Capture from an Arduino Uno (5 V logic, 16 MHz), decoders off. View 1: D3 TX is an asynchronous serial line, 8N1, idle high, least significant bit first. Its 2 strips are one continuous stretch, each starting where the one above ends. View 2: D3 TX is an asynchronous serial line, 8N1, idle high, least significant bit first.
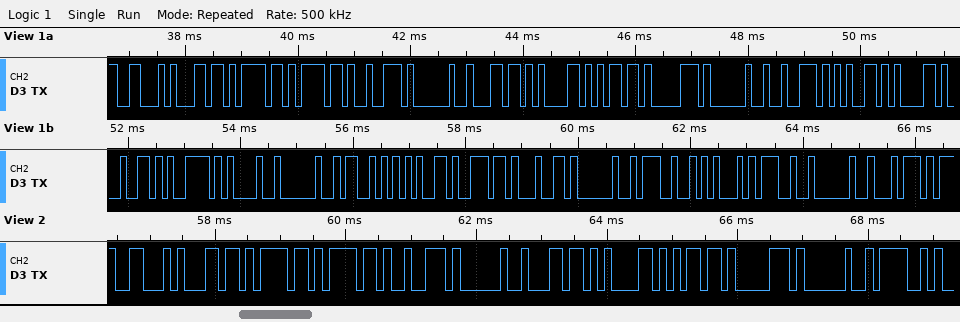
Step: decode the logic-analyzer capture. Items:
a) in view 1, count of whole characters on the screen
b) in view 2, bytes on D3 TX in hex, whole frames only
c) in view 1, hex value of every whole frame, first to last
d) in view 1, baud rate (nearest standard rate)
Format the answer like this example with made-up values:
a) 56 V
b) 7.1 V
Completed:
a) 28
b) 46 6C 6F 6F 72 20 6C 61 6D 70 20 4F
c) 46 6C 6F 6F 72 20 6C 61 6D 70 20 72 65 61 64 79 21 20 53 65 6E 64 20 27 45 27 20 74
d) 9600 baud
